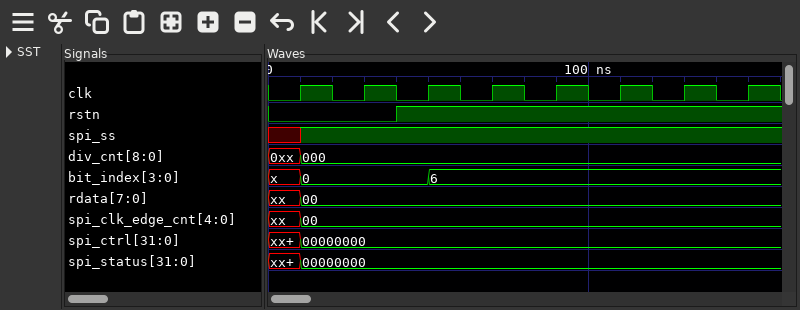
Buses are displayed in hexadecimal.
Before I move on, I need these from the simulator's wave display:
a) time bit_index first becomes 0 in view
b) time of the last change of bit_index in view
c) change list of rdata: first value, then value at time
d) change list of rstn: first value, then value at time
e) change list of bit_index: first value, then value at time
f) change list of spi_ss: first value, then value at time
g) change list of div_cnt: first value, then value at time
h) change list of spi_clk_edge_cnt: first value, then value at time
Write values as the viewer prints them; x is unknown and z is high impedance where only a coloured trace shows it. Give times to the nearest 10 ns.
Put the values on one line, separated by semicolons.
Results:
10 ns; 50 ns; xx, 00 at 10 ns; 0, 1 at 40 ns; x, 0 at 10 ns, 6 at 50 ns; x, 1 at 10 ns; 0xx, 000 at 10 ns; xx, 00 at 10 ns
